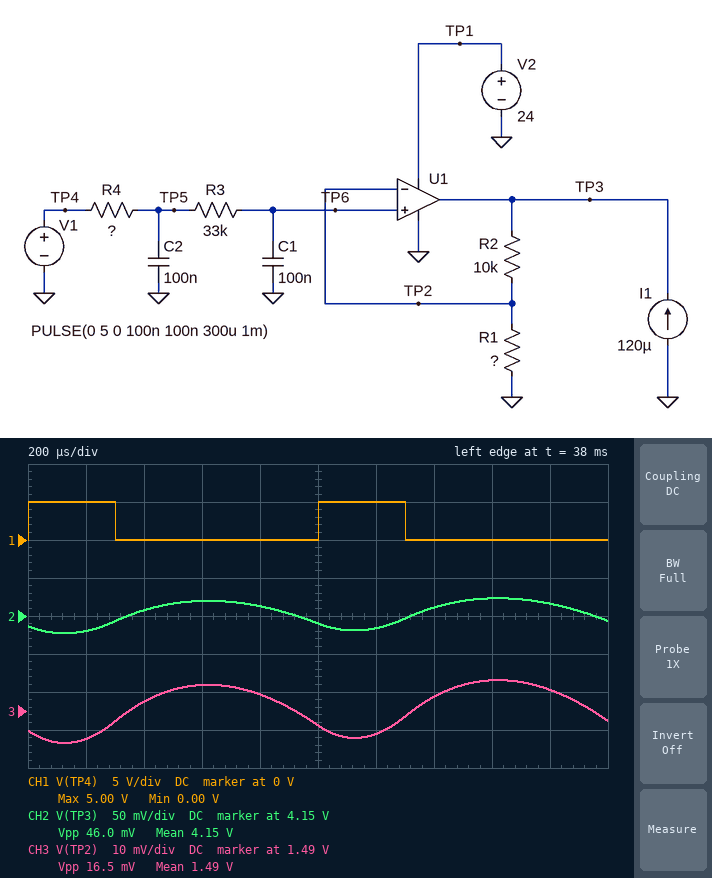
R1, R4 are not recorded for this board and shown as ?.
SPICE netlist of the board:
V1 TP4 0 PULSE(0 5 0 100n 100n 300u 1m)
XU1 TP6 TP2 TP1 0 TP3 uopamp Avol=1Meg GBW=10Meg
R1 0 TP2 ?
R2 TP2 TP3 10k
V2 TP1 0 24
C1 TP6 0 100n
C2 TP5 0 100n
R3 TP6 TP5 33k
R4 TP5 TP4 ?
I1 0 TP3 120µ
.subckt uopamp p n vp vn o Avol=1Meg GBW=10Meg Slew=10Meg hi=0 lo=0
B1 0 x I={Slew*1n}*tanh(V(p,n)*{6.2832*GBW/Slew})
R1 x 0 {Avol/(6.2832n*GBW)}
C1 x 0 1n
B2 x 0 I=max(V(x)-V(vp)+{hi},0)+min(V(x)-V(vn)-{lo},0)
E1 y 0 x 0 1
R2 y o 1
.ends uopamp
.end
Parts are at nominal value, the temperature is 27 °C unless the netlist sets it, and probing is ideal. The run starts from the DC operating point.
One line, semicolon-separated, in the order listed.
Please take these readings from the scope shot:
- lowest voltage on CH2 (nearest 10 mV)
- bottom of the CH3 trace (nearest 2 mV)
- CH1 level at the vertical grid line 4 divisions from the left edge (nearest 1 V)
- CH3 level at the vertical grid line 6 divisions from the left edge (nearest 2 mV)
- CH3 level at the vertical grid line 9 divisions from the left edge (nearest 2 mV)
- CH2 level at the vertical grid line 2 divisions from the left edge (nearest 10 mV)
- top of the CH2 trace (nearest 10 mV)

4.13 V; 1.482 V; 0 V; 1.484 V; 1.496 V; 4.16 V; 4.17 V
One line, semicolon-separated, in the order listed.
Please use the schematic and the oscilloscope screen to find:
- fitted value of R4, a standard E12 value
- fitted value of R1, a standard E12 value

27 kΩ; 5.6 kΩ
